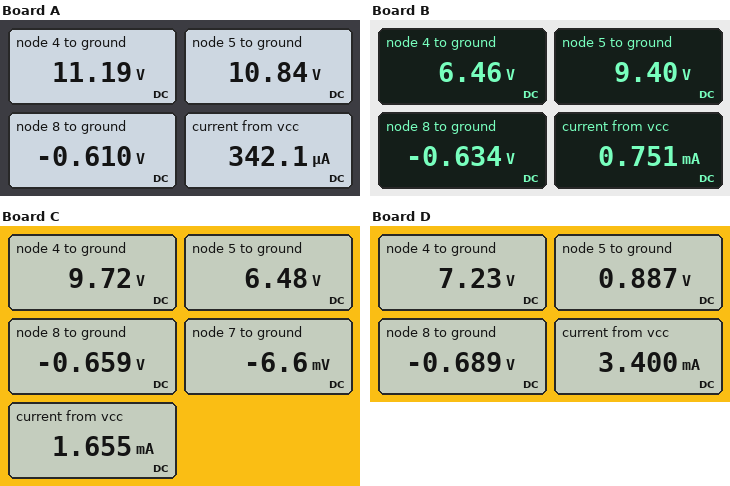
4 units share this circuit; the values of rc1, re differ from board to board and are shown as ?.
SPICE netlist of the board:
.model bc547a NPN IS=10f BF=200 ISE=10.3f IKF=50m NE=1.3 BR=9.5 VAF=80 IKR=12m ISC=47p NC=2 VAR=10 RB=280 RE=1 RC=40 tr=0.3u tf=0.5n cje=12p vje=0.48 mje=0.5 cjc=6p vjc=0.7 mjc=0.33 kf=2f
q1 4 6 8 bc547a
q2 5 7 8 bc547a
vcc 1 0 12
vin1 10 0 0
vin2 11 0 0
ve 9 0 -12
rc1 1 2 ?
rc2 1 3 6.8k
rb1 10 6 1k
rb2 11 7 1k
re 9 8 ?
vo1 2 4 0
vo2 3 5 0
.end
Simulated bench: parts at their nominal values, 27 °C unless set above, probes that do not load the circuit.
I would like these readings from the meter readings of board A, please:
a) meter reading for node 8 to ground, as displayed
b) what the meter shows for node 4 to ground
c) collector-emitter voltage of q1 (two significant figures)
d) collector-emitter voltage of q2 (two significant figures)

-0.610 V
11.19 V
12 V
11 V
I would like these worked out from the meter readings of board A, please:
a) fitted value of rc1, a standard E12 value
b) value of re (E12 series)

4.7 kΩ
33 kΩ
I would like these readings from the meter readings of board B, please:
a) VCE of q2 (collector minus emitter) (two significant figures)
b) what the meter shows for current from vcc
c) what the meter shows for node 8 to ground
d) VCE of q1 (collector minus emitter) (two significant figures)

10 V
0.751 mA
-0.634 V
7.1 V
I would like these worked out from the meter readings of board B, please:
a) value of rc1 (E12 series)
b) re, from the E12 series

15 kΩ
15 kΩ
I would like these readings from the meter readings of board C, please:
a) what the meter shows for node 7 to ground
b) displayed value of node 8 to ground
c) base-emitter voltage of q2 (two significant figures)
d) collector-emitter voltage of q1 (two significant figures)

-6.6 mV
-0.659 V
650 mV
10 V
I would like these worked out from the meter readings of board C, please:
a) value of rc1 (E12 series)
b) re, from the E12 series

2.7 kΩ
6.8 kΩ
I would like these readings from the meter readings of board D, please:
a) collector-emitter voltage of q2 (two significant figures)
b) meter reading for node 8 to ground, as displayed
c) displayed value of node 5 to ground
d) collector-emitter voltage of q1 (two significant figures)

1.6 V
-0.689 V
0.887 V
7.9 V
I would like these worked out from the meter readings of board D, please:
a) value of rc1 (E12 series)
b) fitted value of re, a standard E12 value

2.7 kΩ
3.3 kΩ
